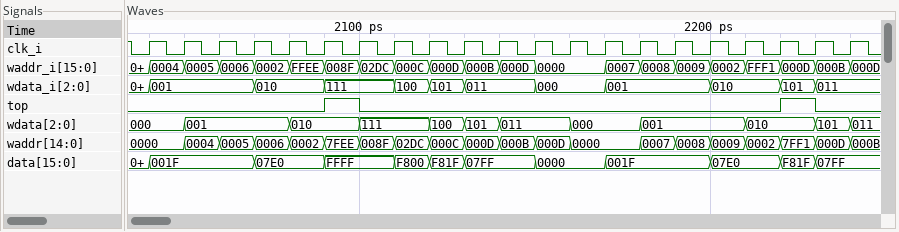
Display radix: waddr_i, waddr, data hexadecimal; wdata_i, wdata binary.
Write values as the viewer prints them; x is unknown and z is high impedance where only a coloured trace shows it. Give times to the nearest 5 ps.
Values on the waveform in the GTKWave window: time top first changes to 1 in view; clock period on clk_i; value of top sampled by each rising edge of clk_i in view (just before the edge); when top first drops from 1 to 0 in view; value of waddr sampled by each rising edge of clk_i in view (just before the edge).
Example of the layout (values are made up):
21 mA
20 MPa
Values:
2090 ps
10 ps
0 0 0 0 0 0 1 0 0 0 0 0 0 0 0 0 0 0 0 1 0
2100 ps
0000, 0000, 0004, 0005, 0006, 0002, 7FEE, 008F, 02DC, 000C, 000D, 000B, 000D, 0000, 0000, 0007, 0008, 0009, 0002, 7FF1, 000D
